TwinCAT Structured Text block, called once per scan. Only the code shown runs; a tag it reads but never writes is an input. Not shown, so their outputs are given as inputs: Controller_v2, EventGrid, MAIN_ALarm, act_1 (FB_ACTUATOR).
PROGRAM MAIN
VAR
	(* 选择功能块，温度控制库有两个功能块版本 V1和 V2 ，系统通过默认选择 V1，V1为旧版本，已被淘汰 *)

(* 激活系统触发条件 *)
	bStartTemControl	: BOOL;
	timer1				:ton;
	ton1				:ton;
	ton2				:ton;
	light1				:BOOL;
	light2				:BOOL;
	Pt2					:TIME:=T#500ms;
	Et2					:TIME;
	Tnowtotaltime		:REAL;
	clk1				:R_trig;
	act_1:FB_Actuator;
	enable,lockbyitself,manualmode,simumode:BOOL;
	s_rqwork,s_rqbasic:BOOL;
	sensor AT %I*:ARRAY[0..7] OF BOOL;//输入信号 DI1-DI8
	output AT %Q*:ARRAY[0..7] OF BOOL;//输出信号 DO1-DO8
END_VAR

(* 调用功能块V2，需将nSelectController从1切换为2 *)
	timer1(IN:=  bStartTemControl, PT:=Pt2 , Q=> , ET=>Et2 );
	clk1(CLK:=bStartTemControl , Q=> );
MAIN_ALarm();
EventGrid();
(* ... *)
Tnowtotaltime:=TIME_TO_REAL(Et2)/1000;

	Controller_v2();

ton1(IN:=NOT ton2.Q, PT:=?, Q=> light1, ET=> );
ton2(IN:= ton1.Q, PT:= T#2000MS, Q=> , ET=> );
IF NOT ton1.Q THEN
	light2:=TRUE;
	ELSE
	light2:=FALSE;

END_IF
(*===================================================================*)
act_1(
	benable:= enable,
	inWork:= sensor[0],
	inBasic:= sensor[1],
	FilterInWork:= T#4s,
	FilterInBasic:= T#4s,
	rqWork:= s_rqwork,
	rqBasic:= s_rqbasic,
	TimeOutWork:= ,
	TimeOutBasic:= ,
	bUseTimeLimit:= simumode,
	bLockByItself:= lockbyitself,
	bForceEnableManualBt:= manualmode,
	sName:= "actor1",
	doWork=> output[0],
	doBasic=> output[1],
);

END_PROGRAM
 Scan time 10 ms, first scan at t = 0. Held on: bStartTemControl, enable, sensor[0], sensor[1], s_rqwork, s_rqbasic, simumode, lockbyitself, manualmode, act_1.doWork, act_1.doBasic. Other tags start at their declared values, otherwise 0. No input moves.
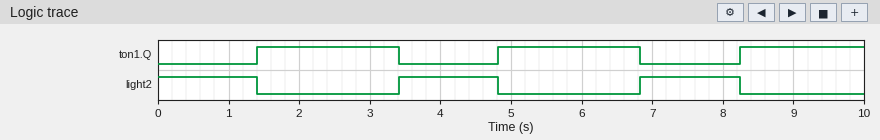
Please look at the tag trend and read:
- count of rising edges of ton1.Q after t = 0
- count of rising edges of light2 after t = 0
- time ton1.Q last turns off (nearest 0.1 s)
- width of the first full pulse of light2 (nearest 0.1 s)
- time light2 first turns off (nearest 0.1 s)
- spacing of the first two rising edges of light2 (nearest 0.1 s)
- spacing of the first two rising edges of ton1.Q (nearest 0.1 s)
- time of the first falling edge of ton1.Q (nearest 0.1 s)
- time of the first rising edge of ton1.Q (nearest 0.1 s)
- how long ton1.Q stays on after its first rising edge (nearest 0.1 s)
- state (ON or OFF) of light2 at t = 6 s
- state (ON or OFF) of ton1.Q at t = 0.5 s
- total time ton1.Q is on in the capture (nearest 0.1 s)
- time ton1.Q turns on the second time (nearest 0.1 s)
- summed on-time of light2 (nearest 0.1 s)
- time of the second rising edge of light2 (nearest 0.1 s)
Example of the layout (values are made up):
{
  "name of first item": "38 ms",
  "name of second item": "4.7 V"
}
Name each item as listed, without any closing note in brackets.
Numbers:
{
  "count of rising edges of ton1.Q after t = 0": "3",
  "count of rising edges of light2 after t = 0": "2",
  "time ton1.Q last turns off": "6.8 s",
  "width of the first full pulse of light2": "1.4 s",
  "time light2 first turns off": "1.4 s",
  "spacing of the first two rising edges of light2": "3.4 s",
  "spacing of the first two rising edges of ton1.Q": "3.4 s",
  "time of the first falling edge of ton1.Q": "3.4 s",
  "time of the first rising edge of ton1.Q": "1.4 s",
  "how long ton1.Q stays on after its first rising edge": "2.0 s",
  "state (ON or OFF) of light2 at t = 6 s": "OFF",
  "state (ON or OFF) of ton1.Q at t = 0.5 s": "OFF",
  "total time ton1.Q is on in the capture": "5.8 s",
  "time ton1.Q turns on the second time": "4.8 s",
  "summed on-time of light2": "4.2 s",
  "time of the second rising edge of light2": "6.8 s"
}
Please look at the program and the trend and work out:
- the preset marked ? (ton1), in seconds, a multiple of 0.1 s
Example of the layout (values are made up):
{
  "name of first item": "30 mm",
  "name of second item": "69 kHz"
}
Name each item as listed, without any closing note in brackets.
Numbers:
{
  "the preset marked ? (ton1), in seconds, a multiple of 0.1 s": "1.4 s"
}
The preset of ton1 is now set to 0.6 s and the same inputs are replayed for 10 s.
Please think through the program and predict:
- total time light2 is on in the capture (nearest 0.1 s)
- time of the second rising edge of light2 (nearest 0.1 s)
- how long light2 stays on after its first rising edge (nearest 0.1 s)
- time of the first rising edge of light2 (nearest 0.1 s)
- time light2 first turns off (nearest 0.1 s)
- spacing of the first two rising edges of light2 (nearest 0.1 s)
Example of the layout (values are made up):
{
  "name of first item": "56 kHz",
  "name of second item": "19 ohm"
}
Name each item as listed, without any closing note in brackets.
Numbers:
{
  "total time light2 is on in the capture": "2.4 s",
  "time of the second rising edge of light2": "5.2 s",
  "how long light2 stays on after its first rising edge": "0.6 s",
  "time of the first rising edge of light2": "2.6 s",
  "time light2 first turns off": "0.6 s",
  "spacing of the first two rising edges of light2": "2.6 s"
}
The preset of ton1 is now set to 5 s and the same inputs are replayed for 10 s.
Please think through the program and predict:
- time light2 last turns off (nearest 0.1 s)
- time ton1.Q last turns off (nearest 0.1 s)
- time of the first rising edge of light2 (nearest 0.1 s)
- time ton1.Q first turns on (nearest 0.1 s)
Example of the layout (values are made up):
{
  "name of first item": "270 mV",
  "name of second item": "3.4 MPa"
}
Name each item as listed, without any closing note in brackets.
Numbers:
{
  "time light2 last turns off": "5.0 s",
  "time ton1.Q last turns off": "7.0 s",
  "time of the first rising edge of light2": "7.0 s",
  "time ton1.Q first turns on": "5.0 s"
}
